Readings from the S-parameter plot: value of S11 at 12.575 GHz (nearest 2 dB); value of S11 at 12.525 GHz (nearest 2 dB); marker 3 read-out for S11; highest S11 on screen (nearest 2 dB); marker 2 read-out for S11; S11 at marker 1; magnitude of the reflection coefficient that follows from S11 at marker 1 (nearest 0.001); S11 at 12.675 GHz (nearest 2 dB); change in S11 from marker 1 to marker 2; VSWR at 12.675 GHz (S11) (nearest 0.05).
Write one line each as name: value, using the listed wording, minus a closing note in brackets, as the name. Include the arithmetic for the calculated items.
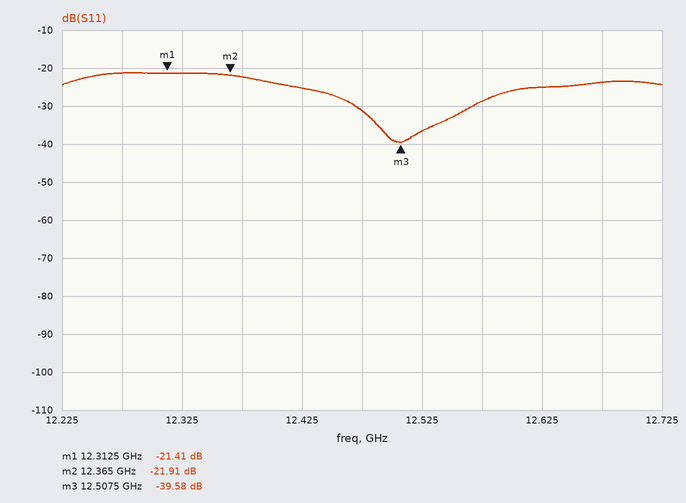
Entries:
value of S11 at 12.575 GHz: -28 dB
value of S11 at 12.525 GHz: -36 dB
marker 3 read-out for S11: -39.58 dB
highest S11 on screen: -22 dB
marker 2 read-out for S11: -21.91 dB
S11 at marker 1: -21.41 dB
magnitude of the reflection coefficient that follows from S11 at marker 1: 10^(-21.41/20) ≈ 0.085
S11 at 12.675 GHz: -24 dB
change in S11 from marker 1 to marker 2: -21.91 − (-21.41) = -0.50 dB
VSWR at 12.675 GHz (S11): |Γ| = 10^(-24/20) = 0.0631; VSWR = (1 + 0.0631)/(1 − 0.0631) ≈ 1.13, so 1.15 to the nearest 0.05
